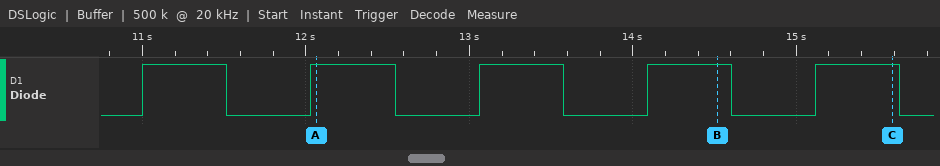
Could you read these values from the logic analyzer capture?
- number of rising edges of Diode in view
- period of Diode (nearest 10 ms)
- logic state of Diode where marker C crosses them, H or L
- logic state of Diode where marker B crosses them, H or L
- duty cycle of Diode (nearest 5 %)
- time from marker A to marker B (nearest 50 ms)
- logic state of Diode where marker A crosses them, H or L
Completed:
5
1030 ms
Diode=H
Diode=H
50 %
2450 ms
Diode=H
